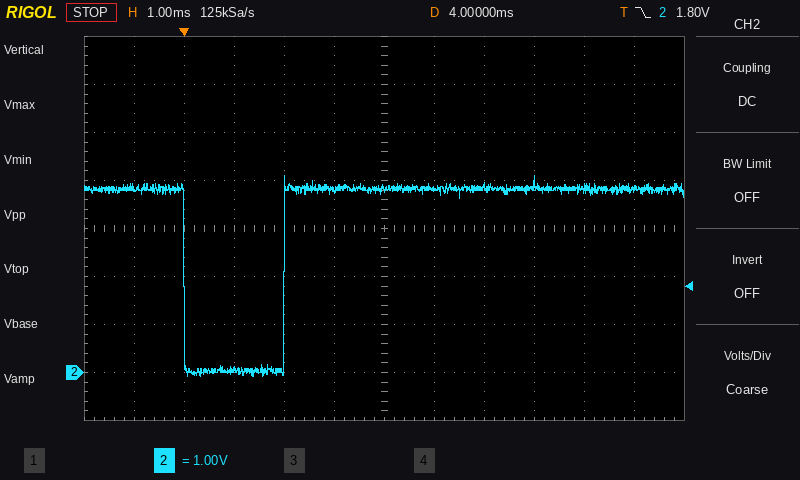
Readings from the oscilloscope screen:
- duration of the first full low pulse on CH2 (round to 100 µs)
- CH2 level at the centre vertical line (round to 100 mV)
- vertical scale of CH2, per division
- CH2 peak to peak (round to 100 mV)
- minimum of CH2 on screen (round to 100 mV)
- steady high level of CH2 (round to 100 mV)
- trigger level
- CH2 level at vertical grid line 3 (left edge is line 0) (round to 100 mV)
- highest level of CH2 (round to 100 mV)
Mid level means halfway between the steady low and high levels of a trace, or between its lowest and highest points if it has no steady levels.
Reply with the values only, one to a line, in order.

2.0 ms
3.8 V
1 V
4.2 V
-100 mV
3.8 V
1.80 V
100 mV
4.1 V
